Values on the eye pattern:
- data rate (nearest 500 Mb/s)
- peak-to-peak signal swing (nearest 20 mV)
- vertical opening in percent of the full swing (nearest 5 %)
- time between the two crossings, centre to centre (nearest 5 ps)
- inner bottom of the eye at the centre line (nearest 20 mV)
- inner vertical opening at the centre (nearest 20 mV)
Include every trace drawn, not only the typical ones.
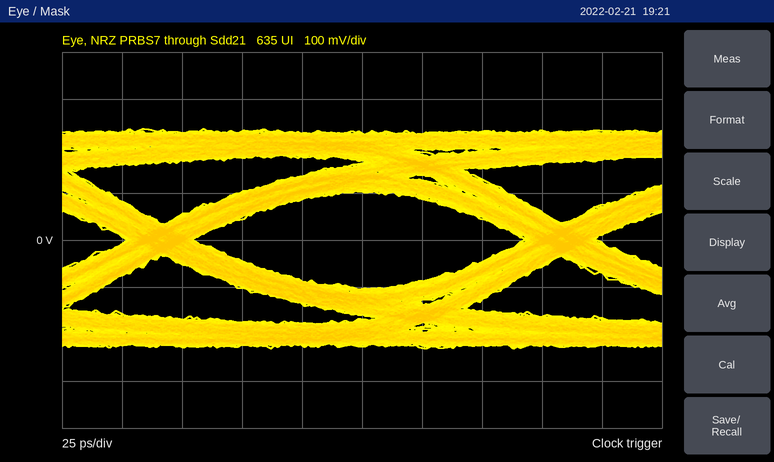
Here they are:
6.0 Gb/s
460 mV
45 %
165 ps
-100 mV
200 mV
